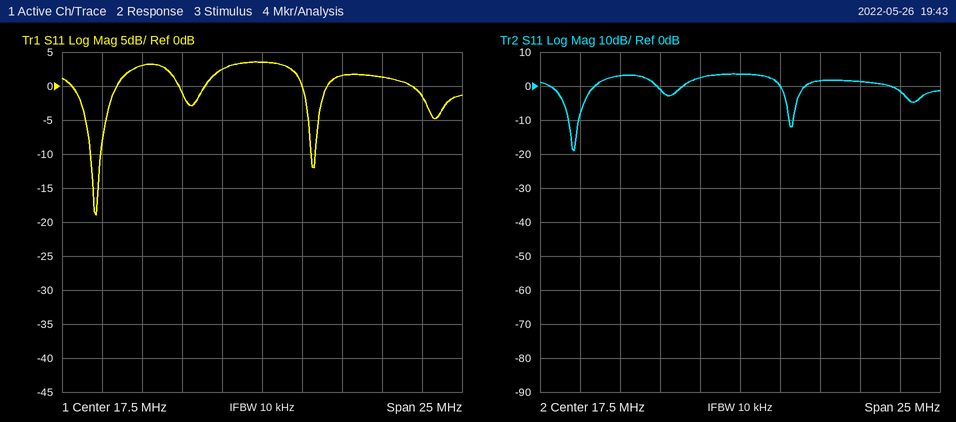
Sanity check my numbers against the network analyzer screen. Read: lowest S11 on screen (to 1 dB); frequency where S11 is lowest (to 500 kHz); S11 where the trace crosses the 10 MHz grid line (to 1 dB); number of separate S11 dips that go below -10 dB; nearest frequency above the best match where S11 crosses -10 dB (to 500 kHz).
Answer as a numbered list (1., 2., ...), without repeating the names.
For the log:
1. -19 dB
2. 7.0 MHz
3. 3 dB
4. 2
5. 7.5 MHz
